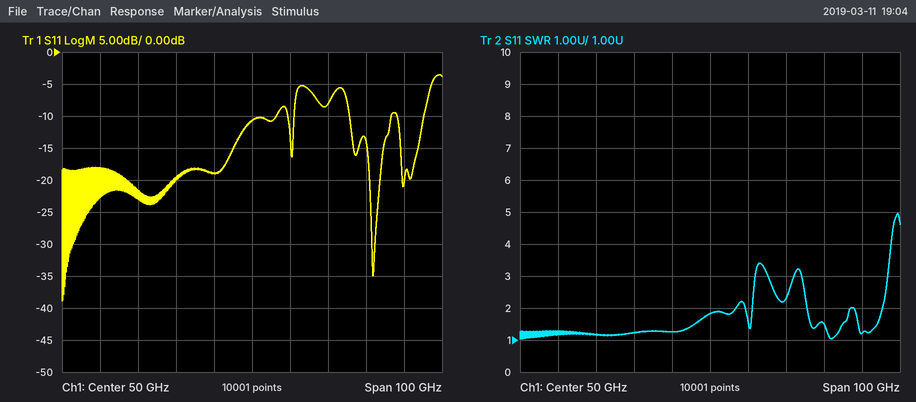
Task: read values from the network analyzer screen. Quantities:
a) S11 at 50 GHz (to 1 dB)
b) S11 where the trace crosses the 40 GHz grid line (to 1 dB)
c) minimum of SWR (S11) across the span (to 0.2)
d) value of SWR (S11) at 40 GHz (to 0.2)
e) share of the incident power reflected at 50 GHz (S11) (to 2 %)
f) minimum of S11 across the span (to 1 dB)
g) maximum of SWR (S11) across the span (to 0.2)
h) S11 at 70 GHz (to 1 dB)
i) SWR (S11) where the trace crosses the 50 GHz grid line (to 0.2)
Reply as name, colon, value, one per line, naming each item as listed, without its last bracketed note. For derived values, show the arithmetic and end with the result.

S11 at 50 GHz: -11 dB
S11 where the trace crosses the 40 GHz grid line: -19 dB
minimum of SWR (S11) across the span: 1.0
value of SWR (S11) at 40 GHz: 1.2
share of the incident power reflected at 50 GHz (S11): 10^(-11/10) ≈ 8 %
minimum of S11 across the span: -39 dB
maximum of SWR (S11) across the span: 5.0
S11 at 70 GHz: -8 dB
SWR (S11) where the trace crosses the 50 GHz grid line: 1.8
